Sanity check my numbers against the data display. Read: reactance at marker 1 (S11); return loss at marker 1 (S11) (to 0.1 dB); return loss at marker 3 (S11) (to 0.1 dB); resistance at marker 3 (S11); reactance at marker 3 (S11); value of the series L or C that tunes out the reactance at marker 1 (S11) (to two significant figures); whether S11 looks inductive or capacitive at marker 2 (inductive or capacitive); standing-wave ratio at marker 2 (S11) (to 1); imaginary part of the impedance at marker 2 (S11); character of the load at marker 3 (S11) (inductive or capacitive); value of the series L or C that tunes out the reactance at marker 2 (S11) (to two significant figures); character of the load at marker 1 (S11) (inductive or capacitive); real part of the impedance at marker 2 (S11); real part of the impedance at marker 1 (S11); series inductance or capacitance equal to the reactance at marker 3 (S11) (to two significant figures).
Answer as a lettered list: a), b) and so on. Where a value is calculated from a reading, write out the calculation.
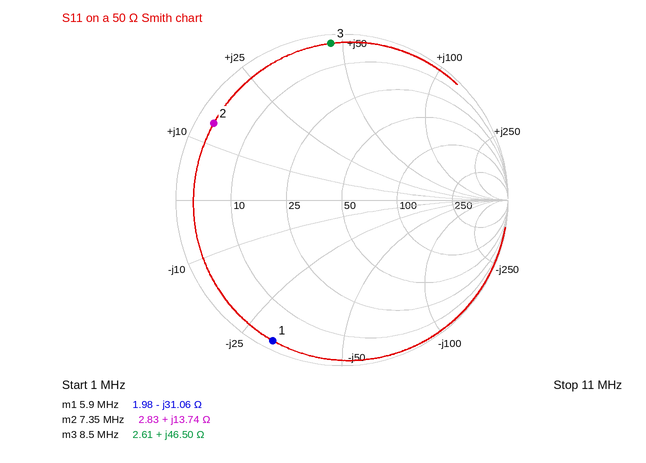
a) -31.06 Ω
b) 0.5 dB
c) 0.5 dB
d) 2.61 Ω
e) +46.50 Ω
f) L = 31.06 Ω/(2π × 5.9 MHz) ≈ 838 nH, so 840 nH to two significant figures
g) inductive
h) 19
i) +13.74 Ω
j) inductive
k) C = 1/(2π × 7.35 MHz × 13.74 Ω) ≈ 1.6 nF
l) capacitive
m) 2.83 Ω
n) 1.98 Ω
o) L = 46.5 Ω/(2π × 8.5 MHz) ≈ 871 nH, so 870 nH to two significant figures
